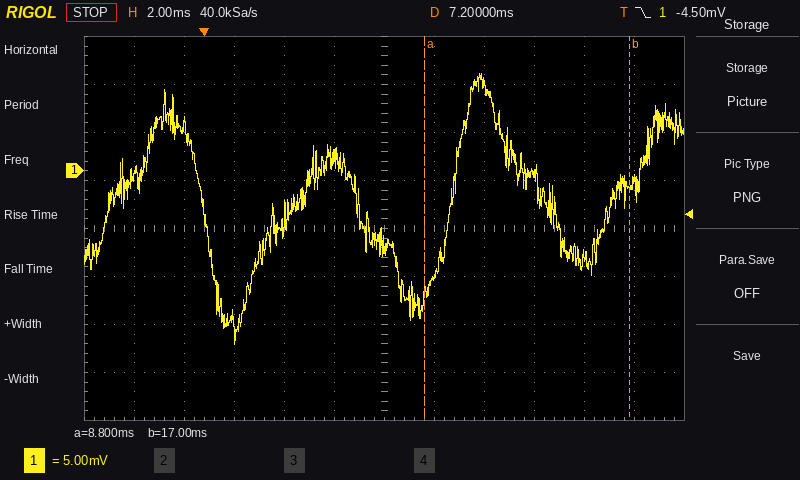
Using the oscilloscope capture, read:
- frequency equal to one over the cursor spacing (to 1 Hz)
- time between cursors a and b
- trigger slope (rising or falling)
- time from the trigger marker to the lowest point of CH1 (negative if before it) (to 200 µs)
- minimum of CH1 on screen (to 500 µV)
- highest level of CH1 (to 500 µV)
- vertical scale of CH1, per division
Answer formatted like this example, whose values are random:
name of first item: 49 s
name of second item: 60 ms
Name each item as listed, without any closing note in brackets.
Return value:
frequency equal to one over the cursor spacing: 122 Hz
time between cursors a and b: 8.2 ms
trigger slope: falling
time from the trigger marker to the lowest point of CH1 (negative if before it): +1.2 ms
minimum of CH1 on screen: -18.0 mV
highest level of CH1: 10.0 mV
vertical scale of CH1, per division: 5 mV
